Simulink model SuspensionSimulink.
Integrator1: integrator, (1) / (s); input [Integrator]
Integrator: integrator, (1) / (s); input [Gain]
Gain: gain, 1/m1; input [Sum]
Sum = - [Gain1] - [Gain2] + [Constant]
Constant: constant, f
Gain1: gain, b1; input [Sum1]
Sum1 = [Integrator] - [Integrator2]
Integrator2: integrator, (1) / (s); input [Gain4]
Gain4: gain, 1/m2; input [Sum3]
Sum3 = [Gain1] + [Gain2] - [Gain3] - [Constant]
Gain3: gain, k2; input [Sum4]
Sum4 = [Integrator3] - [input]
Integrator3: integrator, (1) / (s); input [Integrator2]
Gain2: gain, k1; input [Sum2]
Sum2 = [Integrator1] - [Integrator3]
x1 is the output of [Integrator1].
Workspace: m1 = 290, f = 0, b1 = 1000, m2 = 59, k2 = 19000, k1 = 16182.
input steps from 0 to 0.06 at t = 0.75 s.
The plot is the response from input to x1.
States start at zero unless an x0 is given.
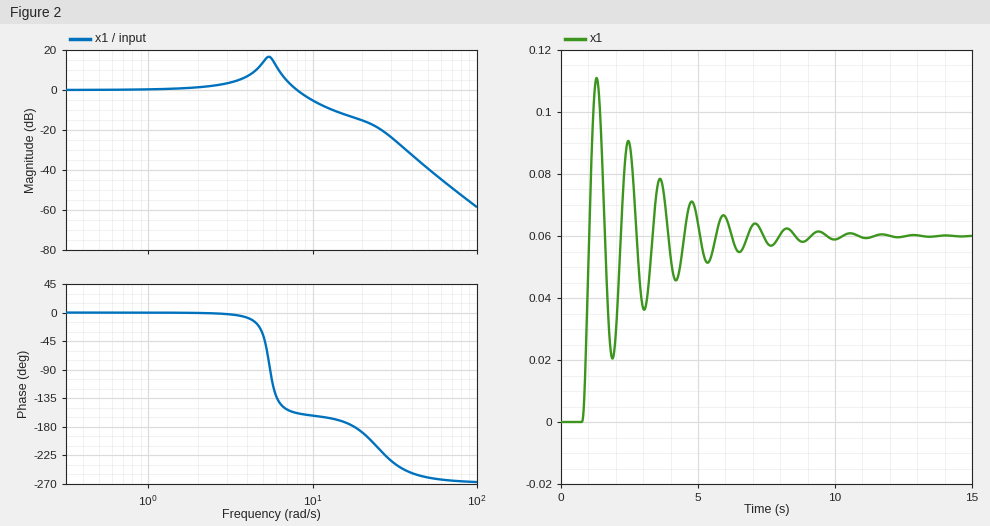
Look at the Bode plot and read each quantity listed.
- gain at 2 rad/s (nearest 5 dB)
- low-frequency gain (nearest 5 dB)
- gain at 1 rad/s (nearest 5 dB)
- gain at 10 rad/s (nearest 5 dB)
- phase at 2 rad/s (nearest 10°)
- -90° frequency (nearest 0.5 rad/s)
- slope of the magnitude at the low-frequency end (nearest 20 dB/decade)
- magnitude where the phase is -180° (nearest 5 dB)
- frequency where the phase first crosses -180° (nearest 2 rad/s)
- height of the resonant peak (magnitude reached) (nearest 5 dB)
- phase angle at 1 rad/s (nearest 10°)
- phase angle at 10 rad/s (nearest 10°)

0 dB
0 dB
0 dB
-5 dB
0°
5.5 rad/s
0 dB/decade
-15 dB
18 rad/s
15 dB
0°
-160°
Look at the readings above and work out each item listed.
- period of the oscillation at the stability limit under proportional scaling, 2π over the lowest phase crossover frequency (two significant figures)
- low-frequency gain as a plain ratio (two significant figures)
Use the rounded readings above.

0.35 s
1.0
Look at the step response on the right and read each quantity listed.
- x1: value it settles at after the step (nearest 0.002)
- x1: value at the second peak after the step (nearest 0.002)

0.060
0.090
